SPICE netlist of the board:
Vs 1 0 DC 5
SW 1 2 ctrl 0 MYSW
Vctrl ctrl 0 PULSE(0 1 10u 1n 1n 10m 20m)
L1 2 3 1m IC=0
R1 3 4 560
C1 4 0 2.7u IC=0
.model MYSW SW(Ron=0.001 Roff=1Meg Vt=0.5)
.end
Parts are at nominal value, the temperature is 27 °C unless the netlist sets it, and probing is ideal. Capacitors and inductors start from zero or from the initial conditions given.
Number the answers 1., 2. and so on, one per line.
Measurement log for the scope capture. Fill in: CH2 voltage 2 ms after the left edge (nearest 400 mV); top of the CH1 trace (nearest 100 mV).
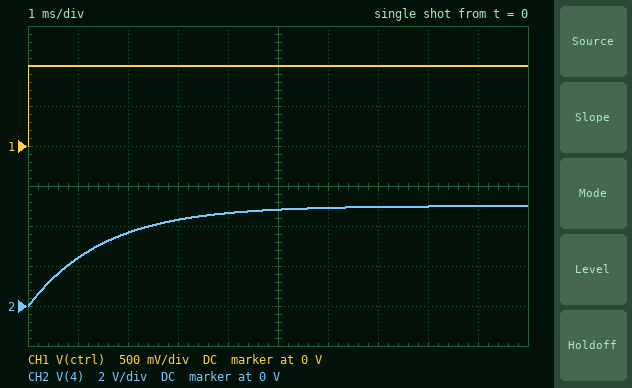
1. 3.6 V
2. 1.0 V
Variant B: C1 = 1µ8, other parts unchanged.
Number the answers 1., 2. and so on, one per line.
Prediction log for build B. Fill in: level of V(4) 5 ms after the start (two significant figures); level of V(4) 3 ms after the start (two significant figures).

1. 5.0 V
2. 4.7 V
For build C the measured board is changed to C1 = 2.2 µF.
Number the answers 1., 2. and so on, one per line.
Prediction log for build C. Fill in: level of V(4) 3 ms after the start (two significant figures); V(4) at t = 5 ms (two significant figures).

1. 4.6 V
2. 4.9 V
